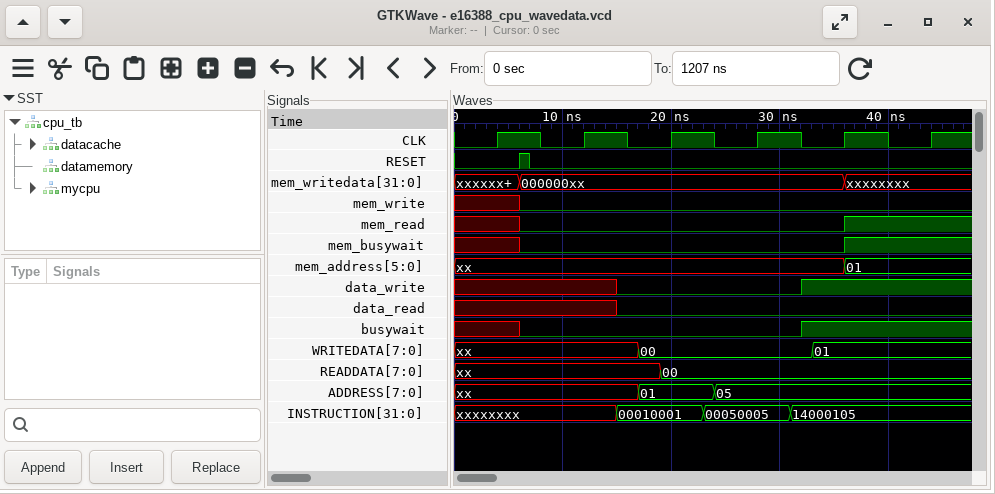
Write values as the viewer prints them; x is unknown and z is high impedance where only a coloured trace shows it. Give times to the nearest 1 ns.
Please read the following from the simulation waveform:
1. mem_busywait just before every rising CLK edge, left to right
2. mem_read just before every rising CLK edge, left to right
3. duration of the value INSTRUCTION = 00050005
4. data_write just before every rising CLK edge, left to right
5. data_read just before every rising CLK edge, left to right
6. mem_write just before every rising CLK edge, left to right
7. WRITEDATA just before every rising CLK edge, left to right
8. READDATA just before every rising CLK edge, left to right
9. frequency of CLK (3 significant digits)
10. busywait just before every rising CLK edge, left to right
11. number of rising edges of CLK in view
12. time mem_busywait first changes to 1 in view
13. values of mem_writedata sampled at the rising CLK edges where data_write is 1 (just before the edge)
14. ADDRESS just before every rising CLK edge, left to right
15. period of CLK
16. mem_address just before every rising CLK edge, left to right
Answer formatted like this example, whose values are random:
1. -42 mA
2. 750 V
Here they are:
1. x 0 0 0 0 1
2. x 0 0 0 0 1
3. 8 ns
4. x x 0 0 1 1
5. x x 0 0 0 0
6. x 0 0 0 0 0
7. xx, xx, 00, 00, 01, 01
8. xx, xx, 00, 00, 00, 00
9. 125 MHz
10. x 0 0 0 1 1
11. 6
12. 36 ns
13. 000000xx, xxxxxxxx
14. xx, xx, 01, 05, 05, 05
15. 8 ns
16. xx, xx, xx, xx, xx, 01
